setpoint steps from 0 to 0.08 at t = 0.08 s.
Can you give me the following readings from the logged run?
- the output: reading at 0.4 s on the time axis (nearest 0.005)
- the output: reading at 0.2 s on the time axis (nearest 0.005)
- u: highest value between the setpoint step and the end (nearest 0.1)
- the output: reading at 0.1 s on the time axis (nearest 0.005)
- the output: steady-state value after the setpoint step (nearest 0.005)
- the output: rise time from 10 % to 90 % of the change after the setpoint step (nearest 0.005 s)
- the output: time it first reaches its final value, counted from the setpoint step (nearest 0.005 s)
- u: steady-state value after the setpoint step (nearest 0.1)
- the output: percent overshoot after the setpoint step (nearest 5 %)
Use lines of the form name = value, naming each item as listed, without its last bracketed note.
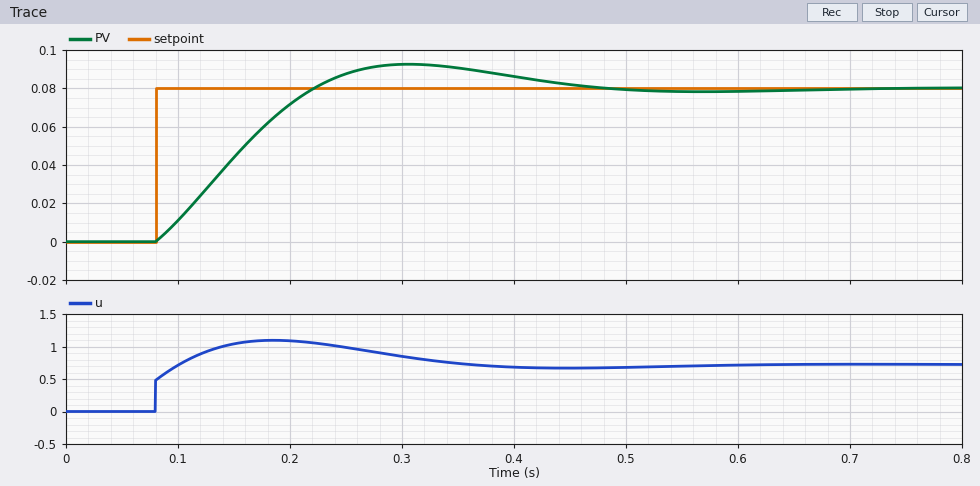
the output: reading at 0.4 s on the time axis = 0.085
the output: reading at 0.2 s on the time axis = 0.070
u: highest value between the setpoint step and the end = 1.1
the output: reading at 0.1 s on the time axis = 0.010
the output: steady-state value after the setpoint step = 0.080
the output: rise time from 10 % to 90 % of the change after the setpoint step = 0.105 s
the output: time it first reaches its final value, counted from the setpoint step = 0.140 s
u: steady-state value after the setpoint step = 0.7
the output: percent overshoot after the setpoint step = 15 %
